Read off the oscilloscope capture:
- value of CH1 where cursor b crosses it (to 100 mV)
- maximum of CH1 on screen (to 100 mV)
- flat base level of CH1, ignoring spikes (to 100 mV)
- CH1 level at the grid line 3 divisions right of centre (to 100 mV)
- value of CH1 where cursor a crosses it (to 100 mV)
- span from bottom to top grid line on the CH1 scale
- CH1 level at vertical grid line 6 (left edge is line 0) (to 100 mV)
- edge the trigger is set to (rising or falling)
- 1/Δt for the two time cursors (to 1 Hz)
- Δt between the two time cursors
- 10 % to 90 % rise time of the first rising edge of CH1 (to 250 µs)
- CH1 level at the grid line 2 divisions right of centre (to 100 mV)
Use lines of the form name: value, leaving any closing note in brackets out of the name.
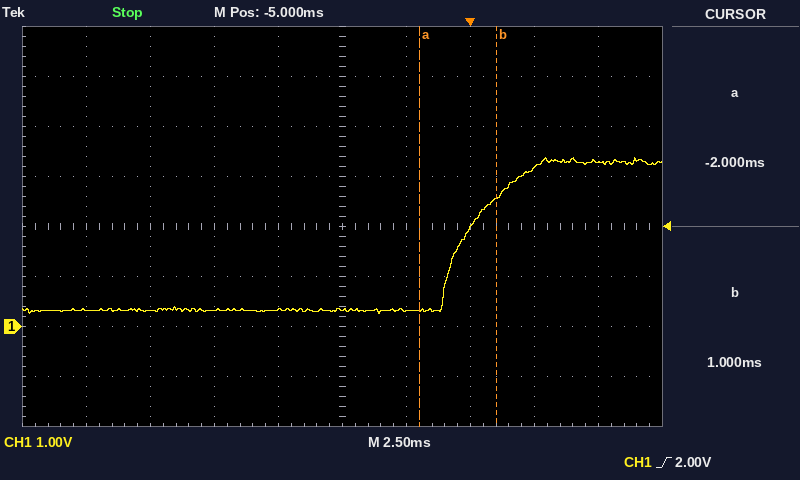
value of CH1 where cursor b crosses it: 2.6 V
maximum of CH1 on screen: 3.4 V
flat base level of CH1, ignoring spikes: 300 mV
CH1 level at the grid line 3 divisions right of centre: 3.2 V
value of CH1 where cursor a crosses it: 300 mV
span from bottom to top grid line on the CH1 scale: 8 V
CH1 level at vertical grid line 6 (left edge is line 0): 300 mV
edge the trigger is set to: rising
1/Δt for the two time cursors: 333 Hz
Δt between the two time cursors: 3.00 ms
10 % to 90 % rise time of the first rising edge of CH1: 3.00 ms
CH1 level at the grid line 2 divisions right of centre: 2.0 V
